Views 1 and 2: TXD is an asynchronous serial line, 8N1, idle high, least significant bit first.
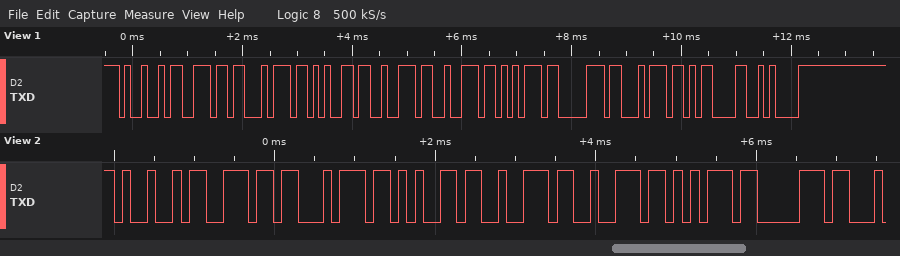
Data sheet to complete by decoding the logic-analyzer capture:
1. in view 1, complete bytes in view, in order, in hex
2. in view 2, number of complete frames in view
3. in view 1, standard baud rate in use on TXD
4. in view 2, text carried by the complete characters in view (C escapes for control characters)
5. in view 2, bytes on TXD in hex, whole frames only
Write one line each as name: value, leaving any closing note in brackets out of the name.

in view 1, complete bytes in view, in order, in hex: 49 6E 74 65 72 72 75 70 74 0D 0A
in view 2, number of complete frames in view: 8
in view 1, standard baud rate in use on TXD: 9600 baud
in view 2, text carried by the complete characters in view: "Interrup"
in view 2, bytes on TXD in hex, whole frames only: 0x49 0x6E 0x74 0x65 0x72 0x72 0x75 0x70
